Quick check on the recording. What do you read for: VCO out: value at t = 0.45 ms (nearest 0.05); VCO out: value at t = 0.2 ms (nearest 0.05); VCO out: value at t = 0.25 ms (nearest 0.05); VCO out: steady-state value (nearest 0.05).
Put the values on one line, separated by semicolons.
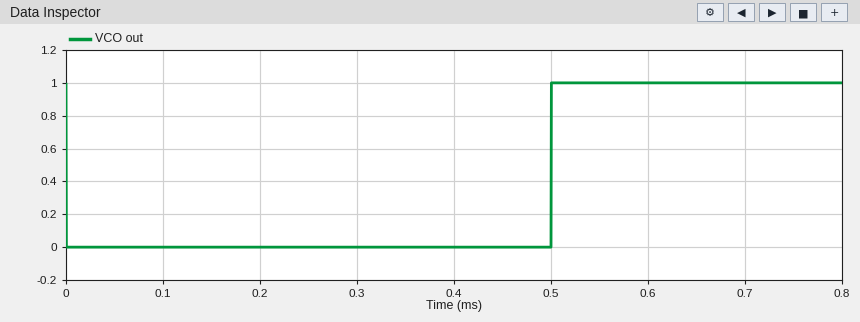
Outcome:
0.00; 0.00; 0.00; 1.00
